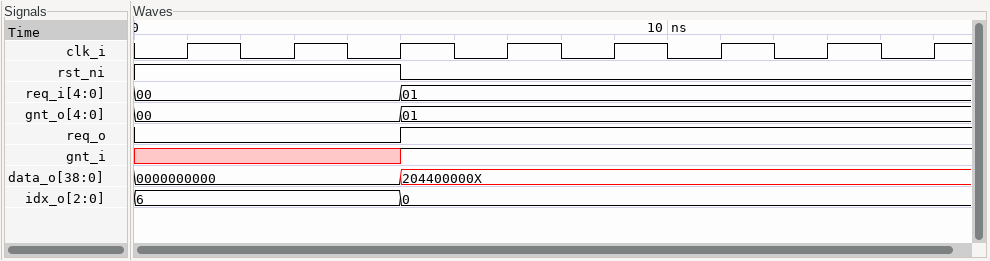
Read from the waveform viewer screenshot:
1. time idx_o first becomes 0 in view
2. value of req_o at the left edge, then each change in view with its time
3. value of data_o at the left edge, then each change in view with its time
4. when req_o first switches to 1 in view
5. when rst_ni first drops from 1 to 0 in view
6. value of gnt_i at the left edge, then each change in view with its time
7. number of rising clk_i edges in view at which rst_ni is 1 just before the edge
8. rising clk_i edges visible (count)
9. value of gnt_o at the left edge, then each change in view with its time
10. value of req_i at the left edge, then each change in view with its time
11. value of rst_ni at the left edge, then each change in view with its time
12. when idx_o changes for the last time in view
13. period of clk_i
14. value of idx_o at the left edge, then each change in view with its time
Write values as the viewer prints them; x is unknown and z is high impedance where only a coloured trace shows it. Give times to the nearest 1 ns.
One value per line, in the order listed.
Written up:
5 ns
0, 1 at 5 ns
0000000000, 204400000X at 5 ns
5 ns
5 ns
x, 1 at 5 ns
3
8
00, 01 at 5 ns
00, 01 at 5 ns
1, 0 at 5 ns
5 ns
2 ns
6, 0 at 5 ns
